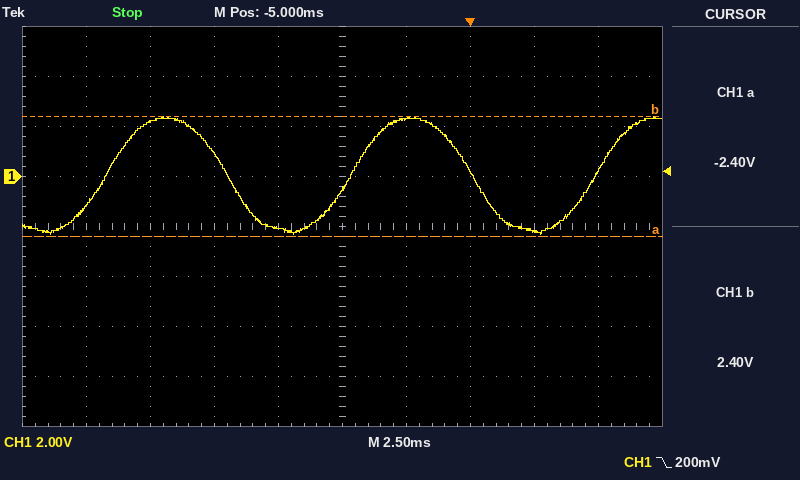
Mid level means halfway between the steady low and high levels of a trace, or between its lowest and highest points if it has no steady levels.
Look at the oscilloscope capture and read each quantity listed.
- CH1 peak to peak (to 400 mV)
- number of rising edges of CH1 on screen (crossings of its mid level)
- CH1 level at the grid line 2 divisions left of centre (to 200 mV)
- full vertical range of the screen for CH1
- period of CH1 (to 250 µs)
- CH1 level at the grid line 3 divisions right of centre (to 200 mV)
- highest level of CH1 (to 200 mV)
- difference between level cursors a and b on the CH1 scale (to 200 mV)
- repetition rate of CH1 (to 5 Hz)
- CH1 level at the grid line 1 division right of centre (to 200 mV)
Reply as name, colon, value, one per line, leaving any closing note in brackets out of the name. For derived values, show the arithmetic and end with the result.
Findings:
CH1 peak to peak: 4.8 V
number of rising edges of CH1 on screen: 3
CH1 level at the grid line 2 divisions left of centre: 1.0 V
full vertical range of the screen for CH1: 16 V
period of CH1: 9.50 ms
CH1 level at the grid line 3 divisions right of centre: -2.2 V
highest level of CH1: 2.4 V
difference between level cursors a and b on the CH1 scale: 4.8 V
repetition rate of CH1: 1 / 9.50 ms ≈ 105 Hz
CH1 level at the grid line 1 division right of centre: 2.4 V
